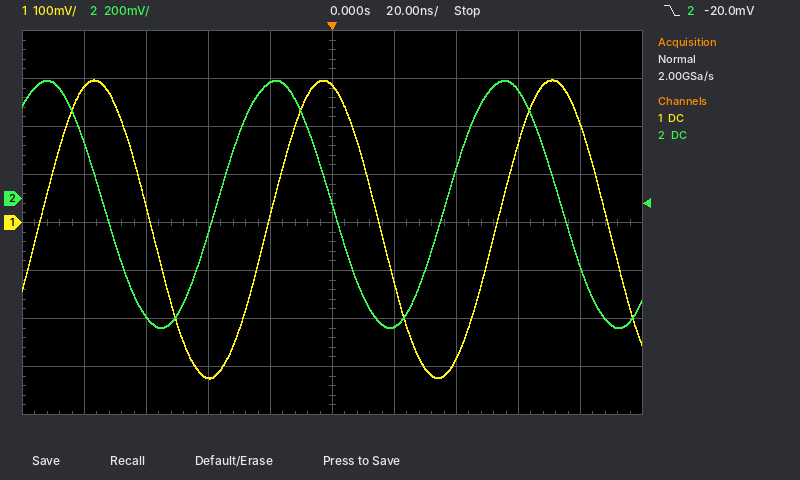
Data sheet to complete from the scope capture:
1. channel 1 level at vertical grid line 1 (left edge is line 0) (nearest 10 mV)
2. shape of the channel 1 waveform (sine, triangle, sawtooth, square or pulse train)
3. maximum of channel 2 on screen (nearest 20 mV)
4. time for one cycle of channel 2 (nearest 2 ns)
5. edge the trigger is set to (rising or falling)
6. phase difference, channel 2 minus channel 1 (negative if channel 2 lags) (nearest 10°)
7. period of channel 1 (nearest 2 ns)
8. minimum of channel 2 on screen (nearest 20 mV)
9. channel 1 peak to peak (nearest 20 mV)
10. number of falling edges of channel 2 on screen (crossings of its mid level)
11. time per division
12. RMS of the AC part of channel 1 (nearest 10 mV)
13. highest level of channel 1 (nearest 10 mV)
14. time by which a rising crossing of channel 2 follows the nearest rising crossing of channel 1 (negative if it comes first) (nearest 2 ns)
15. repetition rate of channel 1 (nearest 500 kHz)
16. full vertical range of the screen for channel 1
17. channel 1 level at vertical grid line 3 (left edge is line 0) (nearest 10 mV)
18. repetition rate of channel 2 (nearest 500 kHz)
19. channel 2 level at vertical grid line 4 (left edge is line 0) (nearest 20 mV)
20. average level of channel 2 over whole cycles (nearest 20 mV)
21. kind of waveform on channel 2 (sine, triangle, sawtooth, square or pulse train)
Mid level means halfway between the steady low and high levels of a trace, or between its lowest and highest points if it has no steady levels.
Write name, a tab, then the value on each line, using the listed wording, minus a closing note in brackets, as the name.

channel 1 level at vertical grid line 1 (left edge is line 0)	280 mV
shape of the channel 1 waveform	sine
maximum of channel 2 on screen	500 mV
time for one cycle of channel 2	74 ns
edge the trigger is set to	falling
phase difference, channel 2 minus channel 1 (negative if channel 2 lags)	+80°
period of channel 1	74 ns
minimum of channel 2 on screen	-540 mV
channel 1 peak to peak	620 mV
number of falling edges of channel 2 on screen	3
time per division	20 ns
RMS of the AC part of channel 1	220 mV
highest level of channel 1	300 mV
time by which a rising crossing of channel 2 follows the nearest rising crossing of channel 1 (negative if it comes first)	-16 ns
repetition rate of channel 1	13.5 MHz
full vertical range of the screen for channel 1	800 mV
channel 1 level at vertical grid line 3 (left edge is line 0)	-320 mV
repetition rate of channel 2	13.5 MHz
channel 2 level at vertical grid line 4 (left edge is line 0)	480 mV
average level of channel 2 over whole cycles	-20 mV
kind of waveform on channel 2	sine
